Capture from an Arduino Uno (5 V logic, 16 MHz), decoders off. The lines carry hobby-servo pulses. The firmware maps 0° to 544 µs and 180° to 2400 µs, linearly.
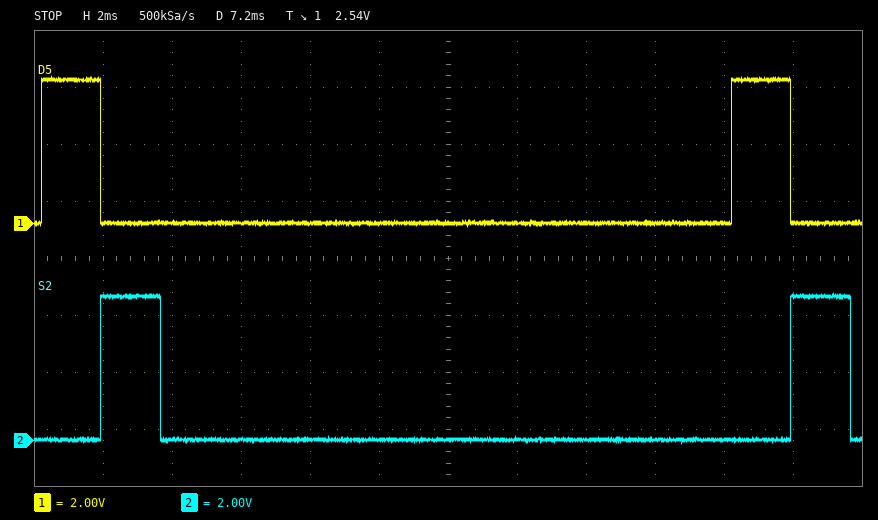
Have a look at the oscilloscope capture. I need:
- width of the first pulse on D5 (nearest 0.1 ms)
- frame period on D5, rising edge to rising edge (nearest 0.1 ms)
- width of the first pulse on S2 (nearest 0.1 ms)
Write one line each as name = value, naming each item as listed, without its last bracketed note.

width of the first pulse on D5 = 1.7 ms
frame period on D5, rising edge to rising edge = 20.0 ms
width of the first pulse on S2 = 1.7 ms
